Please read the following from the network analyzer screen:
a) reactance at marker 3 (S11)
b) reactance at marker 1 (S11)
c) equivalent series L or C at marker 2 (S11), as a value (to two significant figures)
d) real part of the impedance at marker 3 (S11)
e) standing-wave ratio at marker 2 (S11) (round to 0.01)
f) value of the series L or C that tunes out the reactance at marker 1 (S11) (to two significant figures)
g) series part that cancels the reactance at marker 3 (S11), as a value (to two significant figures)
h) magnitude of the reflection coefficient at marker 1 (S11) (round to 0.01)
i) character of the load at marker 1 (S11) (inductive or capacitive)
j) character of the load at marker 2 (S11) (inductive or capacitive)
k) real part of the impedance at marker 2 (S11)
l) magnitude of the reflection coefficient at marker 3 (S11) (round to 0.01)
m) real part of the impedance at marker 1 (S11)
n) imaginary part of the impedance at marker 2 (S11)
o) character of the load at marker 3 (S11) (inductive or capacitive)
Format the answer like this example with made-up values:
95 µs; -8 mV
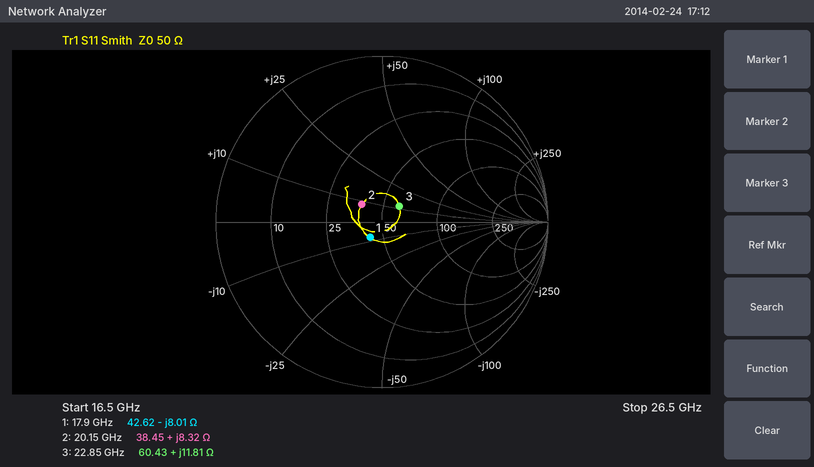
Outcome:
+11.81 Ω; -8.01 Ω; 66 pH; 60.43 Ω; 1.38; 71 pH; 590 fF; 0.12; capacitive; inductive; 38.45 Ω; 0.14; 42.62 Ω; +8.32 Ω; inductive
